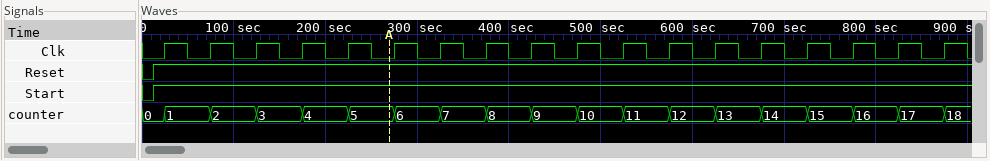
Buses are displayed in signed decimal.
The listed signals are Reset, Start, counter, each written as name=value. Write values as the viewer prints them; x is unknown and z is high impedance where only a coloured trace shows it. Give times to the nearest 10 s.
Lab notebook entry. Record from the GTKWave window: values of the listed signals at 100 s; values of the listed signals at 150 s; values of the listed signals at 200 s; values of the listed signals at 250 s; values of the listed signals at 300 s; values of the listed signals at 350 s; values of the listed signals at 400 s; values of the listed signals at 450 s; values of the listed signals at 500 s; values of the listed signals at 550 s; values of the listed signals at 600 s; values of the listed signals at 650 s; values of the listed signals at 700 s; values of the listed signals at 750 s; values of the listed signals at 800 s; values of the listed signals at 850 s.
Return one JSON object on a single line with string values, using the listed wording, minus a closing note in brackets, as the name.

{"values of the listed signals at 100 s": "Reset=1, Start=1, counter=2", "values of the listed signals at 150 s": "Reset=1, Start=1, counter=3", "values of the listed signals at 200 s": "Reset=1, Start=1, counter=4", "values of the listed signals at 250 s": "Reset=1, Start=1, counter=5", "values of the listed signals at 300 s": "Reset=1, Start=1, counter=6", "values of the listed signals at 350 s": "Reset=1, Start=1, counter=7", "values of the listed signals at 400 s": "Reset=1, Start=1, counter=8", "values of the listed signals at 450 s": "Reset=1, Start=1, counter=9", "values of the listed signals at 500 s": "Reset=1, Start=1, counter=10", "values of the listed signals at 550 s": "Reset=1, Start=1, counter=11", "values of the listed signals at 600 s": "Reset=1, Start=1, counter=12", "values of the listed signals at 650 s": "Reset=1, Start=1, counter=13", "values of the listed signals at 700 s": "Reset=1, Start=1, counter=14", "values of the listed signals at 750 s": "Reset=1, Start=1, counter=15", "values of the listed signals at 800 s": "Reset=1, Start=1, counter=16", "values of the listed signals at 850 s": "Reset=1, Start=1, counter=17"}
